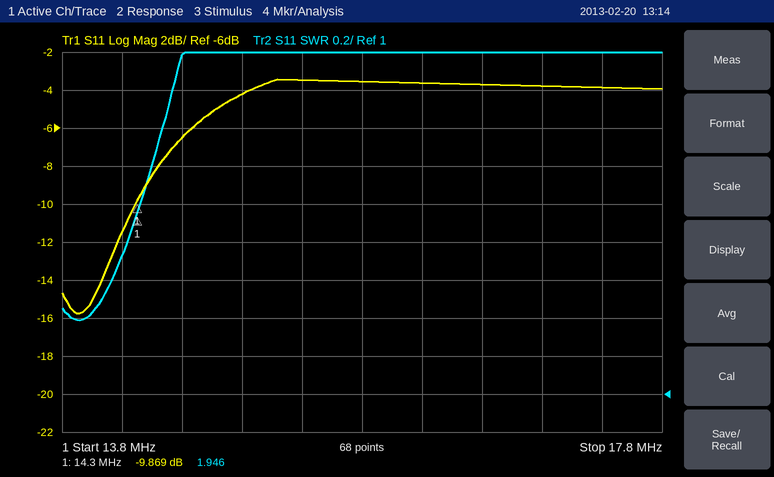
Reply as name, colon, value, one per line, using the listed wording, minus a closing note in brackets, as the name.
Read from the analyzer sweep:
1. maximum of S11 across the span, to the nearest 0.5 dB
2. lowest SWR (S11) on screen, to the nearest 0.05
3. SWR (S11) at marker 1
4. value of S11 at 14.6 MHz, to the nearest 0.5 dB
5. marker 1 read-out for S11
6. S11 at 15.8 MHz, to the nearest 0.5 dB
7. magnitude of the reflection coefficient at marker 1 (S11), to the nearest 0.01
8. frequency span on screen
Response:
maximum of S11 across the span, to the nearest 0.5 dB: -3.5 dB
lowest SWR (S11) on screen, to the nearest 0.05: 1.40
SWR (S11) at marker 1: 1.946
value of S11 at 14.6 MHz, to the nearest 0.5 dB: -6.5 dB
marker 1 read-out for S11: -9.869 dB
S11 at 15.8 MHz, to the nearest 0.5 dB: -3.5 dB
magnitude of the reflection coefficient at marker 1 (S11), to the nearest 0.01: 0.32
frequency span on screen: 4 MHz
